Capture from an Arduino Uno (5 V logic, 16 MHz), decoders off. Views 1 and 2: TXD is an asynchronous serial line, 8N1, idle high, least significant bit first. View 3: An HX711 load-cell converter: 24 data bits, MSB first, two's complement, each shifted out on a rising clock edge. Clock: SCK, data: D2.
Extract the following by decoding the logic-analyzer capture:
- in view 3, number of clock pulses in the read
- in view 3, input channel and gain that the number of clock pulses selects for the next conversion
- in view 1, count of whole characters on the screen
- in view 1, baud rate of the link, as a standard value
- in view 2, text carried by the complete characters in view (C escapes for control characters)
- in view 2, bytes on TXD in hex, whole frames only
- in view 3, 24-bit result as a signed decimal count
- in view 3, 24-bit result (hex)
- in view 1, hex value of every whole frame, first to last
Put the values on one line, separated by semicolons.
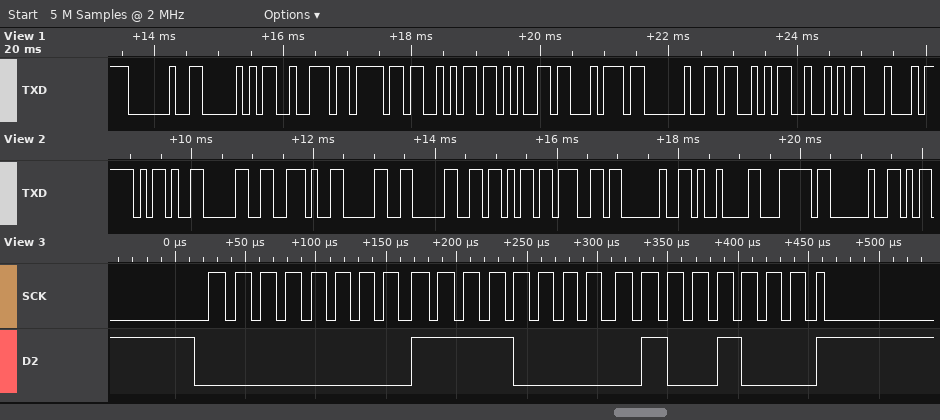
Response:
25; channel A, gain 128; 11; 9600 baud; "-0.00kg \t| "; 2D 30 2E 30 30 6B 67 20 09 7C 20; 61512; 0x00F048; 20 50 72 6F 6A 65 74 20 53 52 44
